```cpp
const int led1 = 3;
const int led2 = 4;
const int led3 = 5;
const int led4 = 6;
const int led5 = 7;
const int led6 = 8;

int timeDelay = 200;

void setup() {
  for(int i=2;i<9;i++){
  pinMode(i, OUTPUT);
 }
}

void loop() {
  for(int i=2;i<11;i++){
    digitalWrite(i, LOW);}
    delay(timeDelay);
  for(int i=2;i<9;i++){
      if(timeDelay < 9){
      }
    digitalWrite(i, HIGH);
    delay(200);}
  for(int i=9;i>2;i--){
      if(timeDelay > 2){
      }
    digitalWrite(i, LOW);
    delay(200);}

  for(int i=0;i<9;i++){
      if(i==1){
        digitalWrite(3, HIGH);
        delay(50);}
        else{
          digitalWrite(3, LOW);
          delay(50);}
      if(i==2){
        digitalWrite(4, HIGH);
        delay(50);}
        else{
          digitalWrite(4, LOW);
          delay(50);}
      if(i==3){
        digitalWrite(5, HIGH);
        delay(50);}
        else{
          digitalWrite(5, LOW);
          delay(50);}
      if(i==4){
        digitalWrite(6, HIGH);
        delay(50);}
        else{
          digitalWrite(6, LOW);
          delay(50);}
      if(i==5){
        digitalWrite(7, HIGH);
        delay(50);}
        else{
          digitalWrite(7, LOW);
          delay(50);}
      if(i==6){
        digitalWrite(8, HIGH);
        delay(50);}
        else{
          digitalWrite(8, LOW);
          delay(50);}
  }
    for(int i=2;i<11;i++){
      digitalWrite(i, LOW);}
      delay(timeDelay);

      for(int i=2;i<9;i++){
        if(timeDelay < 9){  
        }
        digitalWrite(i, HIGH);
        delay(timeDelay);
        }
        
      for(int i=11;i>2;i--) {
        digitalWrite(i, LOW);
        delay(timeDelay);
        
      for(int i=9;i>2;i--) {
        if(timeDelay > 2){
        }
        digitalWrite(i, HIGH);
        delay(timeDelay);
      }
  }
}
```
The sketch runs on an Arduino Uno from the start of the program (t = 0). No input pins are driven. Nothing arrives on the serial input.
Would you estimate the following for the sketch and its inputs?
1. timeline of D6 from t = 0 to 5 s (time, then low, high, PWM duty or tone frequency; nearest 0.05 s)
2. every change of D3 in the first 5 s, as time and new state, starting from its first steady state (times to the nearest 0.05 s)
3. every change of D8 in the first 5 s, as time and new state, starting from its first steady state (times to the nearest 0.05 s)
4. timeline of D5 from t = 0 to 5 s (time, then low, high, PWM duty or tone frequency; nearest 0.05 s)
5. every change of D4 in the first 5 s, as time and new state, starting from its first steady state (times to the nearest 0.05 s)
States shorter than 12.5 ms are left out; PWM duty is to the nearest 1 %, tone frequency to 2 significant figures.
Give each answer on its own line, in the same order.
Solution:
0 s low; 1 s high; 2.2 s low; 4.35 s high; 4.65 s low
0 s low; 0.4 s high; 2.8 s low; 3.3 s high; 3.6 s low
0 s low; 1.4 s high; 1.8 s low
0 s low; 0.8 s high; 2.4 s low; 4 s high; 4.3 s low
0 s low; 0.6 s high; 2.6 s low; 3.65 s high; 3.95 s low
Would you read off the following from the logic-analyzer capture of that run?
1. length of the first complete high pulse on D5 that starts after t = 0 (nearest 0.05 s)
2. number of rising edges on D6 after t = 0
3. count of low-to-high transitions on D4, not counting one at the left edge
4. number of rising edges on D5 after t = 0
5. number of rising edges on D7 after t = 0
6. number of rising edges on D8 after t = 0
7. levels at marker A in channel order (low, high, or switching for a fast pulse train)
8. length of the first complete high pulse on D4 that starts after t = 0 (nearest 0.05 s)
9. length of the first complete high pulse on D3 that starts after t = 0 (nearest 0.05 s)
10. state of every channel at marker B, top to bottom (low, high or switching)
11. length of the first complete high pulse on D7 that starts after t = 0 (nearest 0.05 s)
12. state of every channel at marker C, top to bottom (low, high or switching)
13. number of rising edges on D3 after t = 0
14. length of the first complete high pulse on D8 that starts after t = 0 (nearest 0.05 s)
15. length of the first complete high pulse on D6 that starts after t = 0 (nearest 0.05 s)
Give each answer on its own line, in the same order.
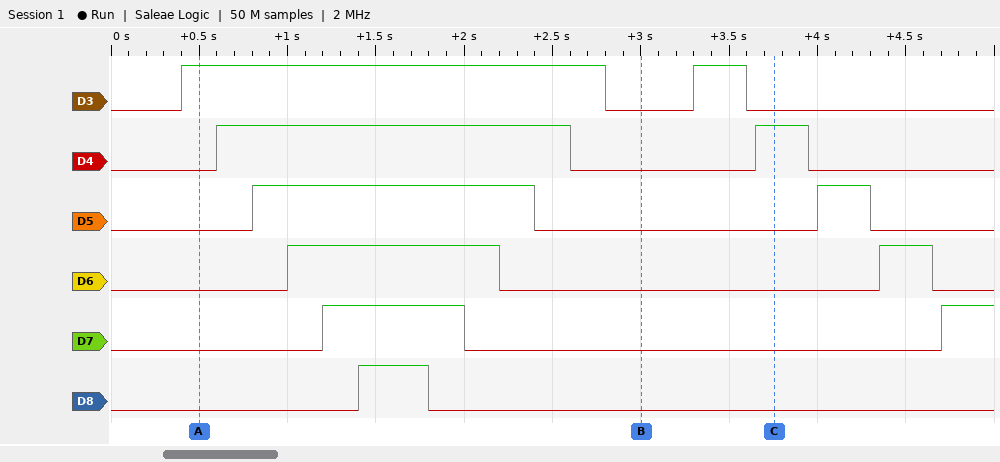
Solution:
1.60 s
2
2
2
2
1
D3 high, D4 low, D5 low, D6 low, D7 low, D8 low
2.00 s
2.40 s
D3 low, D4 low, D5 low, D6 low, D7 low, D8 low
0.80 s
D3 low, D4 high, D5 low, D6 low, D7 low, D8 low
2
0.40 s
1.20 s
